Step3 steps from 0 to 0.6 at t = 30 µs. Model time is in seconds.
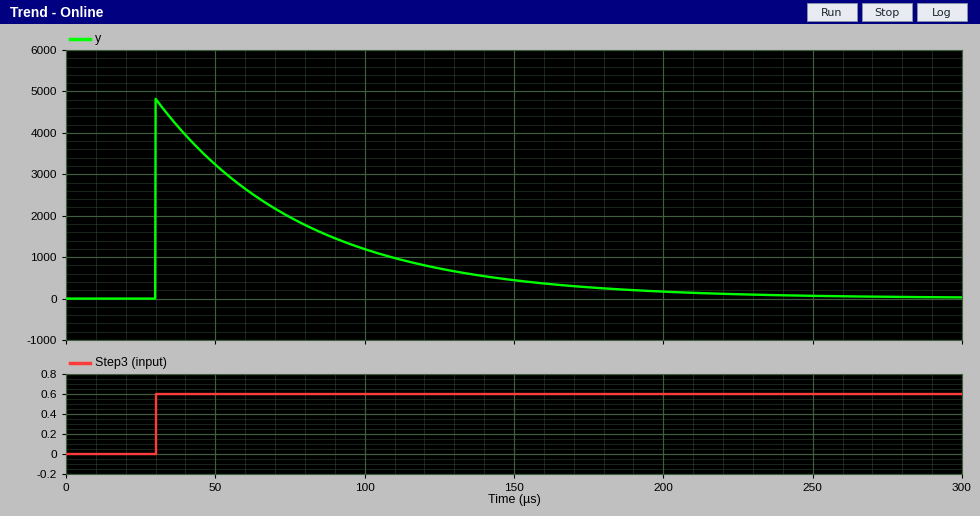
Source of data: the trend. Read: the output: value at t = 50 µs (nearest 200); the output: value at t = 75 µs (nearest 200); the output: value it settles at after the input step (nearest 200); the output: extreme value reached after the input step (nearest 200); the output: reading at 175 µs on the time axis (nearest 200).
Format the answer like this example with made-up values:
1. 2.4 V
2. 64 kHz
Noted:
1. 3200
2. 2000
3. 0
4. 4800
5. 200
